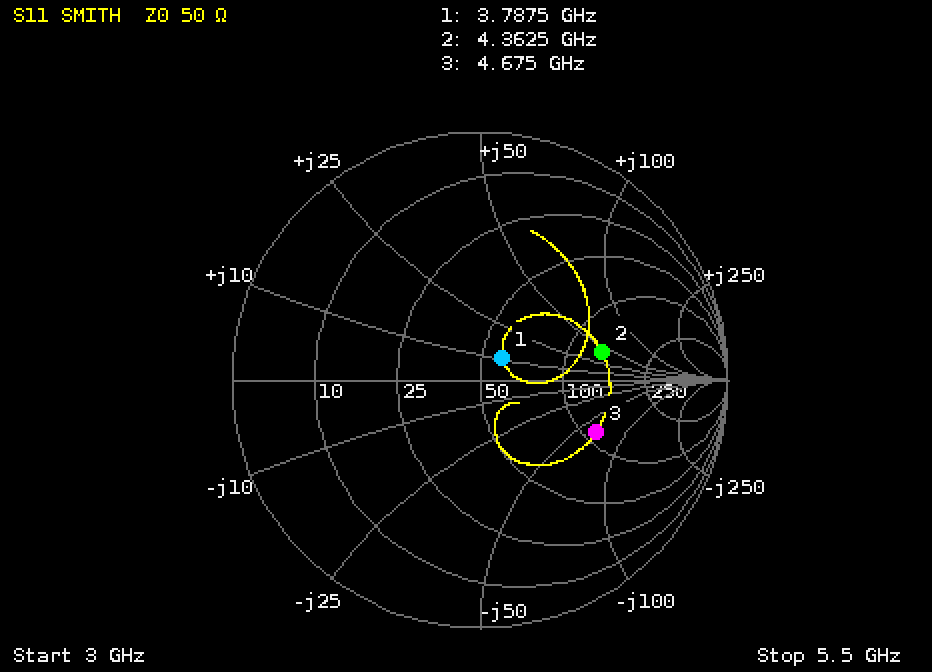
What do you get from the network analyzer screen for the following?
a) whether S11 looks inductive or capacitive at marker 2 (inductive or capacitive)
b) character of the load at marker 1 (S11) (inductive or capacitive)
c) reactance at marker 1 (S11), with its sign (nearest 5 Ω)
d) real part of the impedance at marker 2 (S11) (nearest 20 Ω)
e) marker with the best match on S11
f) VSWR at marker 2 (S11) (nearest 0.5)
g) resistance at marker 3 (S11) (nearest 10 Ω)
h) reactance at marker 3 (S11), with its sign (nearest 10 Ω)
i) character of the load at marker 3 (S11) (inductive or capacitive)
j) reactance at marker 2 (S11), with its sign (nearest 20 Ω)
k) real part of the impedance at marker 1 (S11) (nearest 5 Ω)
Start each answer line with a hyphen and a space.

- inductive
- inductive
- +10 Ω
- 140 Ω
- marker 1
- 3.0
- 110 Ω
- -60 Ω
- capacitive
- +40 Ω
- 60 Ω
